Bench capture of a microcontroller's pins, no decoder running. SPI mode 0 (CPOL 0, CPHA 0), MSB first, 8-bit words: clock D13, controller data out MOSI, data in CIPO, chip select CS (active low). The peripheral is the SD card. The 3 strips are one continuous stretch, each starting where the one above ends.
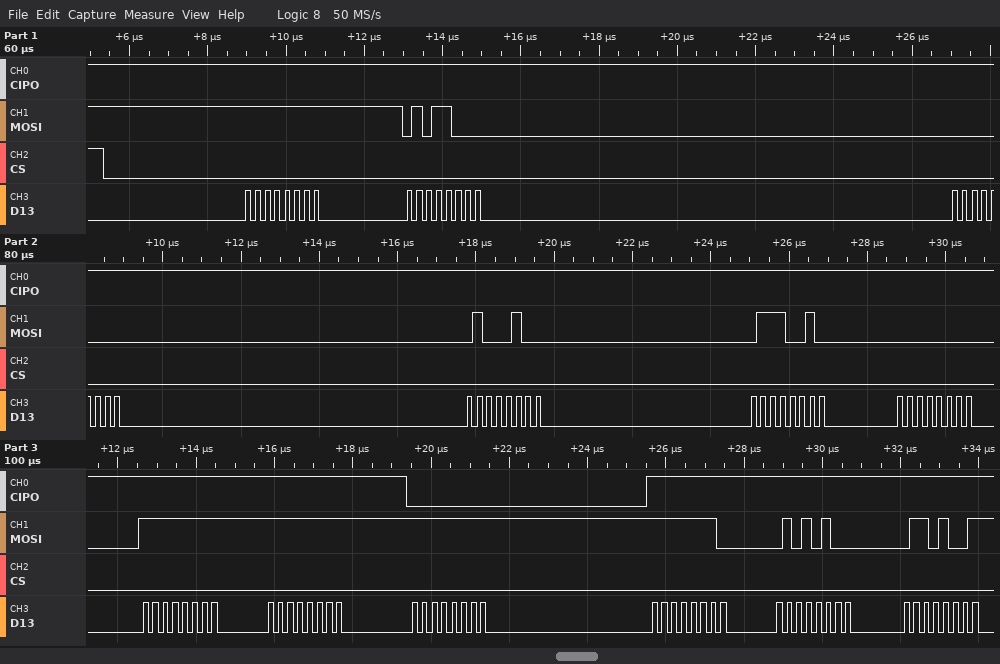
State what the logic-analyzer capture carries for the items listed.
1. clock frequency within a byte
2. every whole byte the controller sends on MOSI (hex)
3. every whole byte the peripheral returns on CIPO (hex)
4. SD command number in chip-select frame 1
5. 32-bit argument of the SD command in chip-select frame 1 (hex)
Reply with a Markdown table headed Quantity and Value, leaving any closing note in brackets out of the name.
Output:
| Quantity | Value |
|---|---|
| clock frequency within a byte | 4 MHz |
| every whole byte the controller sends on MOSI | FF 58 00 44 72 00 FF FF FF FE 54 69 |
| every whole byte the peripheral returns on CIPO | FF FF FF FF FF FF FF FF 00 FF FF FF |
| SD command number in chip-select frame 1 | CMD24 |
| 32-bit argument of the SD command in chip-select frame 1 | 0x00447200 |
